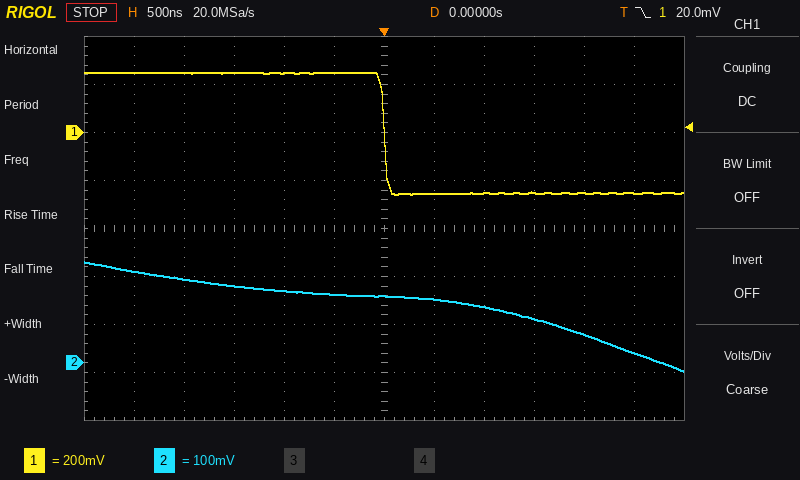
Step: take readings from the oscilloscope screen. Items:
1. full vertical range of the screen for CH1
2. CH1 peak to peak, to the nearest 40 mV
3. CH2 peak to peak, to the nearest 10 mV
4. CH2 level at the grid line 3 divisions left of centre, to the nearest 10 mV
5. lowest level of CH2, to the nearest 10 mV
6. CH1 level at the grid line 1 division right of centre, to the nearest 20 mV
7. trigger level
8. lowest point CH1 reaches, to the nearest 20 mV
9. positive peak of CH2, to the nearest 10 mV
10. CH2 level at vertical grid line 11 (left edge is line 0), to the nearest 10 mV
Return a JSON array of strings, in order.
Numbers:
["1.6 V", "520 mV", "230 mV", "160 mV", "-20 mV", "-260 mV", "20.0 mV", "-260 mV", "210 mV", "20 mV"]
